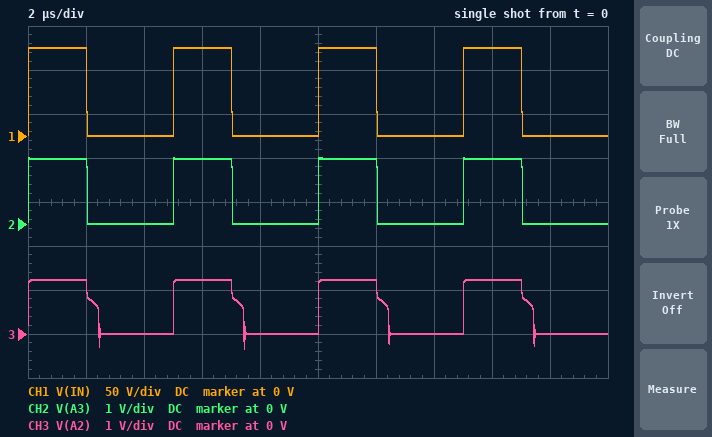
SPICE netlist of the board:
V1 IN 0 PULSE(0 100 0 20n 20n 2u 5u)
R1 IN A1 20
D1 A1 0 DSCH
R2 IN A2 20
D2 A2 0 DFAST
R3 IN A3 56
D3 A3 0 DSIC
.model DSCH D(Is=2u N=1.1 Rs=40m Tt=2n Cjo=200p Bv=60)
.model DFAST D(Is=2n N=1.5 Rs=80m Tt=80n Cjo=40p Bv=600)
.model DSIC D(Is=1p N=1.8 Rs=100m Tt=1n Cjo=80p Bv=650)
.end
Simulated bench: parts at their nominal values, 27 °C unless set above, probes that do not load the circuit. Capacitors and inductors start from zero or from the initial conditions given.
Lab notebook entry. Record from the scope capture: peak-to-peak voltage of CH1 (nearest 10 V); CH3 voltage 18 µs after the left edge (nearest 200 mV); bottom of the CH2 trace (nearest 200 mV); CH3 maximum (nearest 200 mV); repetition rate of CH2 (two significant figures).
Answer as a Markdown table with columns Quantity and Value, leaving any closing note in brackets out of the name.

| Quantity | Value |
|---|---|
| peak-to-peak voltage of CH1 | 100 V |
| CH3 voltage 18 µs after the left edge | 0 V |
| bottom of the CH2 trace | 0 V |
| CH3 maximum | 1.2 V |
| repetition rate of CH2 | 200 kHz |
